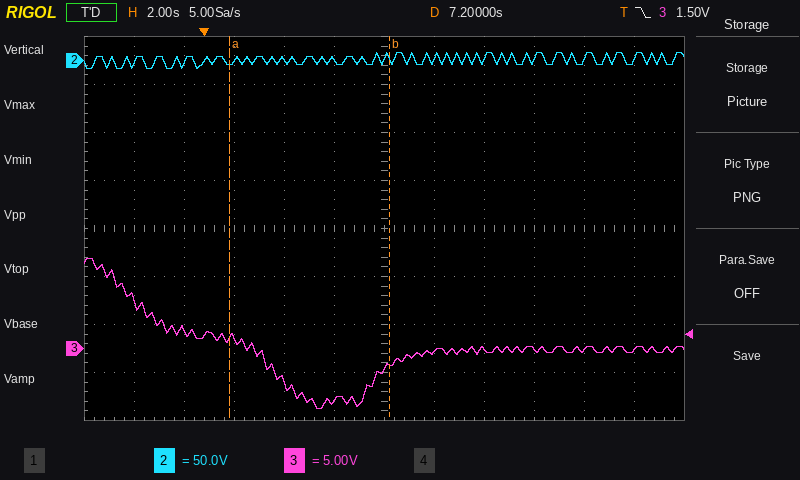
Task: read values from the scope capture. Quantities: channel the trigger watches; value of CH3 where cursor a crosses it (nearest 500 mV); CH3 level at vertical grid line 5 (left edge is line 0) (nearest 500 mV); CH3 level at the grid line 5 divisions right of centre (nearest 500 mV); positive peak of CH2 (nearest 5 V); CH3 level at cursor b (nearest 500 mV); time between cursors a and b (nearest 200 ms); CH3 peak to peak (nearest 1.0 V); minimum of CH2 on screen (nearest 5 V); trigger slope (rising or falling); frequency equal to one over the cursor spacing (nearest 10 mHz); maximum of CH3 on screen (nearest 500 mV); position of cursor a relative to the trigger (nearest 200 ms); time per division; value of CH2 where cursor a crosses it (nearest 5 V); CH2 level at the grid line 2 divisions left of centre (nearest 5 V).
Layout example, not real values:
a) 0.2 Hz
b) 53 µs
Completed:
a) CH3
b) 1.0 V
c) -5.5 V
d) 0.0 V
e) 10 V
f) -1.5 V
g) 6.4 s
h) 16.0 V
i) -10 V
j) falling
k) 160 mHz
l) 9.5 V
m) +1.0 s
n) 2 s
o) -5 V
p) 0 V
